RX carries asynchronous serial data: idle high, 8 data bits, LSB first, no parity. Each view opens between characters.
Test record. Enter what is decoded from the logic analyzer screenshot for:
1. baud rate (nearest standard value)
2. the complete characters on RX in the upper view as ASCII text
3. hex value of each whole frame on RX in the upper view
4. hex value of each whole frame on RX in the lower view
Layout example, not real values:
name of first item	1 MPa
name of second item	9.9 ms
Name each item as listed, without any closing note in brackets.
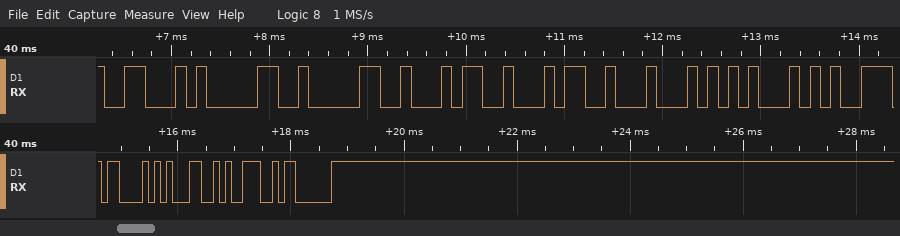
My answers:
baud rate	9600 baud
the complete characters on RX in the upper view as ASCII text	"F0044DE"
hex value of each whole frame on RX in the upper view	46, 30, 30, 34, 34, 44, 45
hex value of each whole frame on RX in the lower view	43, 31, 39, 03
